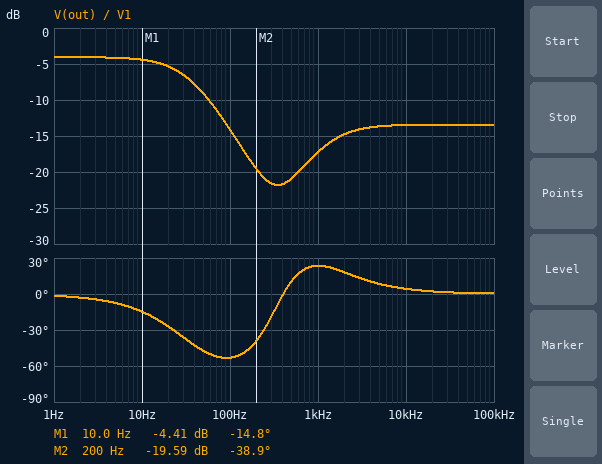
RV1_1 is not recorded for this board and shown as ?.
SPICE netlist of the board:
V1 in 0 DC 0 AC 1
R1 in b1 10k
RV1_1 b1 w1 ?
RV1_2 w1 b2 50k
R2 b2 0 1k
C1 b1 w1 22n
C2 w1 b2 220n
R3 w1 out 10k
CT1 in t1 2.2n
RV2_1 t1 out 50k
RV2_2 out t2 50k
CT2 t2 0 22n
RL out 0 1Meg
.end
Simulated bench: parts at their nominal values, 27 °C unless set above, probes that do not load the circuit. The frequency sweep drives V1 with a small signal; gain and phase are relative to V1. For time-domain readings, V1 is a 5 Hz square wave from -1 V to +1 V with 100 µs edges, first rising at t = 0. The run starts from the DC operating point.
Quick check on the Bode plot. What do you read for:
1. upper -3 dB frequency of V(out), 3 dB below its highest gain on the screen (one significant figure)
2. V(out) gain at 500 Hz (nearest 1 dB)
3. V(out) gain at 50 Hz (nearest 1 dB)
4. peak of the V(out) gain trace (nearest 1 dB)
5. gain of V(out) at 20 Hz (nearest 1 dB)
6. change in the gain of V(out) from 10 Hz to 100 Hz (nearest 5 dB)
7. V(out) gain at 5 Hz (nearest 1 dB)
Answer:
30 Hz
-21 dB
-9 dB
-4 dB
-5 dB
-10 dB
-4 dB
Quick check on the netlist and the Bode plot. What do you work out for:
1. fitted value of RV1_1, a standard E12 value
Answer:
18 kΩ
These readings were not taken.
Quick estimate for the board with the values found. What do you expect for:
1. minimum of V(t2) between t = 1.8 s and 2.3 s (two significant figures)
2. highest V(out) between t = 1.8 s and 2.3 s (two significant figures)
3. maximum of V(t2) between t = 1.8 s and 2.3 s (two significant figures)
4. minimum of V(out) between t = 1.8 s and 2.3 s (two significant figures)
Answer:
-630 mV
630 mV
630 mV
-630 mV
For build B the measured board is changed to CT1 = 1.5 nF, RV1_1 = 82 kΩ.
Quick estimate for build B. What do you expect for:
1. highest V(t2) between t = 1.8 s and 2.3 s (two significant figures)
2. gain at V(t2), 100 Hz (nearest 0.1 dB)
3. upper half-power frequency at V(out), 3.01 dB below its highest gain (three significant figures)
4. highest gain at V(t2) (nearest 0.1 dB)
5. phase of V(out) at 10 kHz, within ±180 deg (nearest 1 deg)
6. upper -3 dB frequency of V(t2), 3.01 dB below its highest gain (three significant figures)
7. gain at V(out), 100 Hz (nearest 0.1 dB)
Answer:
340 mV
-22.2 dB
20.0 Hz
-9.3 dB
6 deg
19.6 Hz
-20.5 dB
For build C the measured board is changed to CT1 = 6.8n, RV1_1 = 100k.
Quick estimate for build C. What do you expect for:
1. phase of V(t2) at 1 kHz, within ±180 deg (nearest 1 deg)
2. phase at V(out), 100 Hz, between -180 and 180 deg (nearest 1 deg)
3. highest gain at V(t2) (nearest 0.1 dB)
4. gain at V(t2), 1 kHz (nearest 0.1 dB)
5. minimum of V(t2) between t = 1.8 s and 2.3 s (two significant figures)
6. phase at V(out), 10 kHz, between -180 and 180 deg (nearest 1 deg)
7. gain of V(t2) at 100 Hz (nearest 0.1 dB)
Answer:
-71 deg
-5 deg
-10.4 dB
-30.9 dB
-300 mV
1 deg
-20.9 dB
